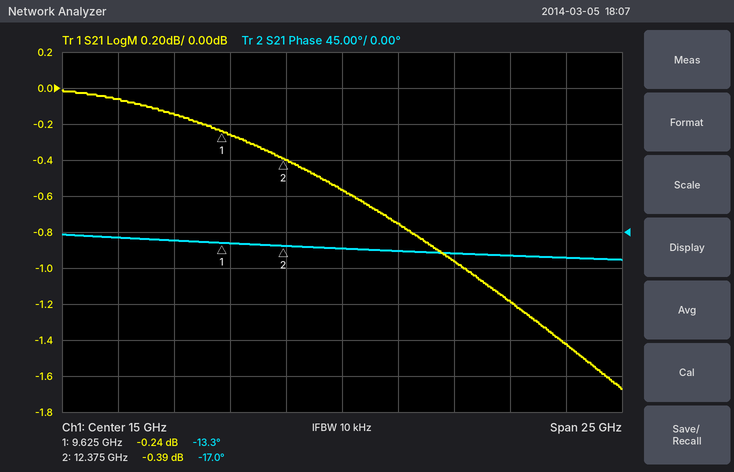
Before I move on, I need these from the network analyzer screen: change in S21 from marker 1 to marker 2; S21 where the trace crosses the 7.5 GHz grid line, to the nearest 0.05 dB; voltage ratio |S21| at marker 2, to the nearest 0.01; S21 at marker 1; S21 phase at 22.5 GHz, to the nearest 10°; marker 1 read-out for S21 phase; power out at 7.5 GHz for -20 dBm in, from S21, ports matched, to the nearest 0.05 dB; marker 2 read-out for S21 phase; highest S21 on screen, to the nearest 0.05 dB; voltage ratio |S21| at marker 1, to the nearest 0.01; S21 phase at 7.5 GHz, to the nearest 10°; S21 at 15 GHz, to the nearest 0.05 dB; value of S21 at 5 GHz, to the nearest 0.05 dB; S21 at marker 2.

-0.15 dB
-0.15 dB
0.96
-0.24 dB
-30°
-13.3°
-20.15 dBm
-17.0°
0.00 dB
0.97
-10°
-0.55 dB
-0.05 dB
-0.39 dB
